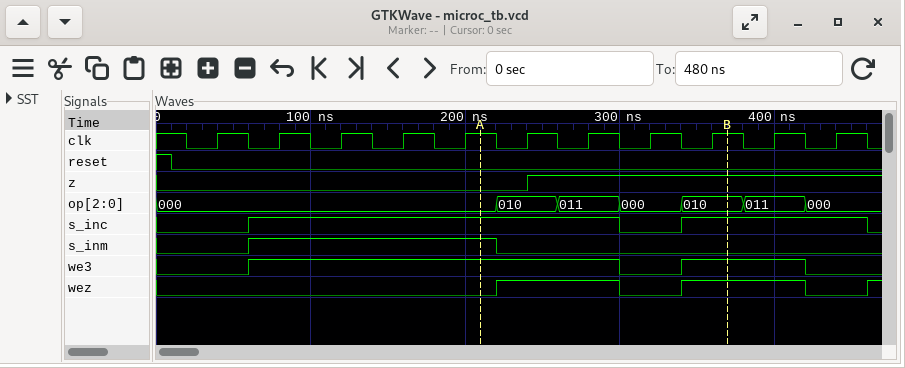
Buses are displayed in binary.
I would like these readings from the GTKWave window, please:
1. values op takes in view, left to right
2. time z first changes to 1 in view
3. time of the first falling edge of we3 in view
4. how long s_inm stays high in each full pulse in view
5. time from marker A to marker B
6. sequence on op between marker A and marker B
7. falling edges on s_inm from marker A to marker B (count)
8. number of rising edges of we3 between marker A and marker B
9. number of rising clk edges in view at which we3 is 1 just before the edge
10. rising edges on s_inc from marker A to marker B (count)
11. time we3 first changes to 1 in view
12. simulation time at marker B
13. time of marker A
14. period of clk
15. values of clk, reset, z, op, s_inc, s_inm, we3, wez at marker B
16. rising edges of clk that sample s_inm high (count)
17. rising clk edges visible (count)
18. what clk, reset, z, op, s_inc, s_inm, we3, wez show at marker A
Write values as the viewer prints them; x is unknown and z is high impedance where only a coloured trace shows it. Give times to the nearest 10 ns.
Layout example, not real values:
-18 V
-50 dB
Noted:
000, 010, 011, 000, 010, 011, 000
240 ns
300 ns
160 ns
160 ns
000, 010, 011, 000, 010
1
1
8
1
60 ns
370 ns
210 ns
40 ns
clk=1, reset=0, z=1, op=010, s_inc=1, s_inm=0, we3=1, wez=1
4
11
clk=1, reset=0, z=0, op=000, s_inc=1, s_inm=1, we3=1, wez=0
